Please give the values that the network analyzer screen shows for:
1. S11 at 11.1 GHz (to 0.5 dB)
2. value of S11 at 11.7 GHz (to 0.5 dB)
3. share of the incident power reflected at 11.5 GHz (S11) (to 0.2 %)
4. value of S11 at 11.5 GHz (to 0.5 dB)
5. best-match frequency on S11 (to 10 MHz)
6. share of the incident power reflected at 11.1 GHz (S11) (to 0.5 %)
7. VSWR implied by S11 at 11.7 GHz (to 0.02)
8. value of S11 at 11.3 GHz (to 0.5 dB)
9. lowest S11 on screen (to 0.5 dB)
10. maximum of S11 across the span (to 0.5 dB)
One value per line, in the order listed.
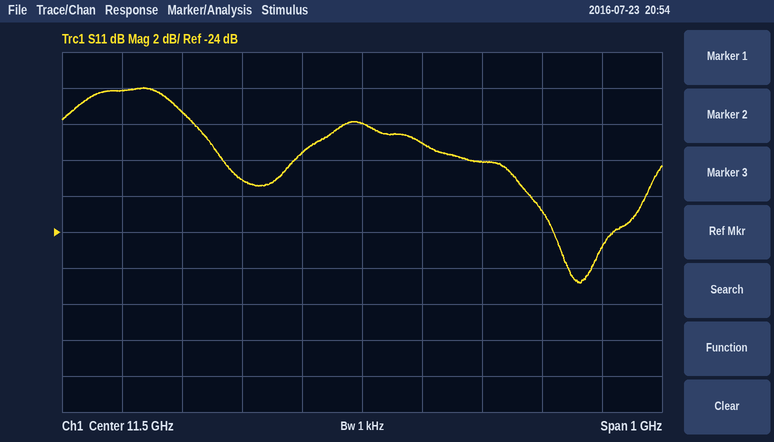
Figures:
-16.0 dB
-20.0 dB
1.6 %
-18.0 dB
11.86 GHz
2.5 %
1.22
-21.0 dB
-27.0 dB
-16.0 dB
